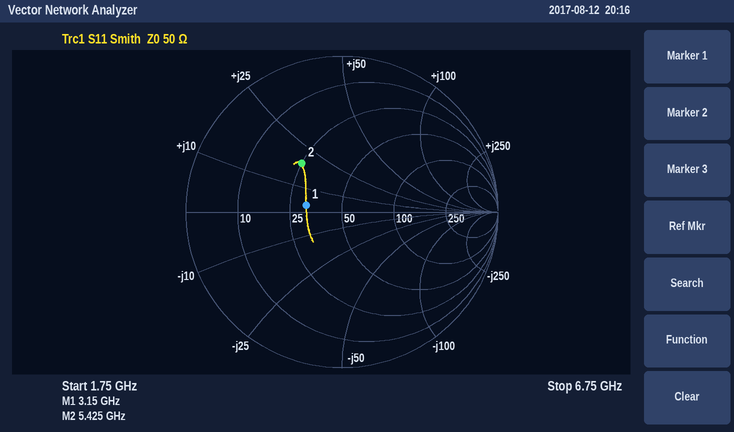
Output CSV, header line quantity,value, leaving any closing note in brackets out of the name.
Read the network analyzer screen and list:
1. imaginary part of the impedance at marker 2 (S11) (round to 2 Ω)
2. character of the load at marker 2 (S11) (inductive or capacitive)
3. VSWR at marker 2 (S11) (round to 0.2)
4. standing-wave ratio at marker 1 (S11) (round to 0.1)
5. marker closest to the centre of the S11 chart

quantity,value
imaginary part of the impedance at marker 2 (S11),+18 Ω
character of the load at marker 2 (S11),inductive
VSWR at marker 2 (S11),2.4
standing-wave ratio at marker 1 (S11),1.6
marker closest to the centre of the S11 chart,marker 1
